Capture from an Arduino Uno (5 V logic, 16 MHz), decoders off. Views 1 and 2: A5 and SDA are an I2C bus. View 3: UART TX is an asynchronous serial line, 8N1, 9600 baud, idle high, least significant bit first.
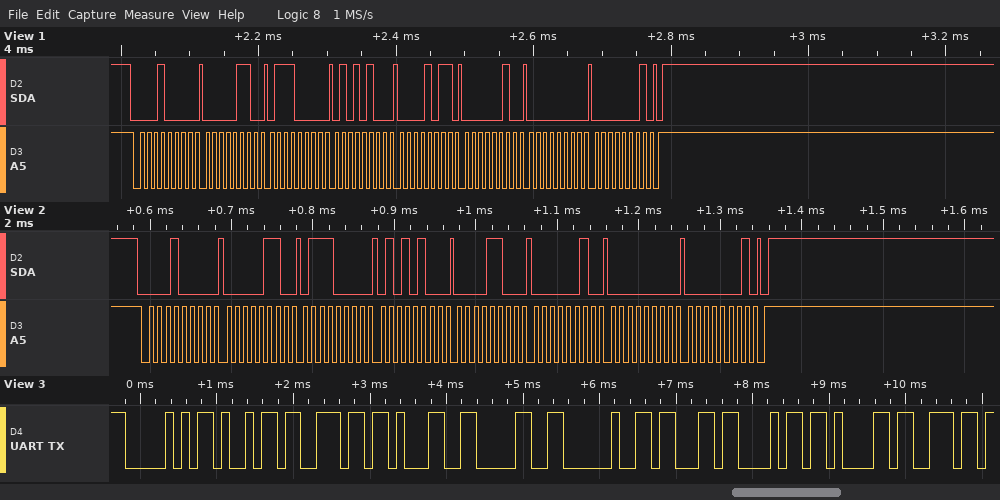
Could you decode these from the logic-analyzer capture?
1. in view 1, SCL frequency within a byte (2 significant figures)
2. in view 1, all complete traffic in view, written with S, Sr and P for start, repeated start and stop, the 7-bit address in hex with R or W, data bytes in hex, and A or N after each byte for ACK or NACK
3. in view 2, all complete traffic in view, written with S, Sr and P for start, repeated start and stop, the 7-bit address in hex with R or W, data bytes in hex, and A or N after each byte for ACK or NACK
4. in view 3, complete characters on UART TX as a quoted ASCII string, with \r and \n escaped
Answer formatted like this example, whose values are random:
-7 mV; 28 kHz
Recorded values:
100 kHz; S 08W A 06 A 70 A 54 A 0B A 02 A 00 A 01 A P; S 08W A 06 A 70 A 54 A 0C A 02 A 00 A 01 A P; "Pin10 chan"
